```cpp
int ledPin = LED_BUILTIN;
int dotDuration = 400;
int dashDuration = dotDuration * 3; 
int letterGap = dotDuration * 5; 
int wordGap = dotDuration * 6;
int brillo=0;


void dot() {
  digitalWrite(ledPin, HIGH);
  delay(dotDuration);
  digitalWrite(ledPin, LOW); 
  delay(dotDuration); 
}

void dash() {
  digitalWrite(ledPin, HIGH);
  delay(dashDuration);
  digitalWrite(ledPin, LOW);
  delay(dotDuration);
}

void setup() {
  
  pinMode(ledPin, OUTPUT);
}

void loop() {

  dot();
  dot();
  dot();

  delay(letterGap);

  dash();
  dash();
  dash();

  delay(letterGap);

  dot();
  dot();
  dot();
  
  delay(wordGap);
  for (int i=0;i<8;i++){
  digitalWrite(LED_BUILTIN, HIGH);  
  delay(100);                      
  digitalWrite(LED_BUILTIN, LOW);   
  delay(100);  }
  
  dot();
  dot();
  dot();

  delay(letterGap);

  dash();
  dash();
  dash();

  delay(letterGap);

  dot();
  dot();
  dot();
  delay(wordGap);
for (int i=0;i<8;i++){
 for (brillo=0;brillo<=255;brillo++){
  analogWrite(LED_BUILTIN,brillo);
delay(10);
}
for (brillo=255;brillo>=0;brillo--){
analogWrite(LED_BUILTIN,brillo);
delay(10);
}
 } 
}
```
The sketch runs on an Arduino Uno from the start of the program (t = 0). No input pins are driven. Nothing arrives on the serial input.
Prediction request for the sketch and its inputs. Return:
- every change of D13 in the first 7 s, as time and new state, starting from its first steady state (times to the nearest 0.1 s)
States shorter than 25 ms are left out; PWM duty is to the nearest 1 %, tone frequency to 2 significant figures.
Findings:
0 s high; 0.4 s low; 0.8 s high; 1.2 s low; 1.6 s high; 2 s low; 4.4 s high; 5.6 s low; 6 s high
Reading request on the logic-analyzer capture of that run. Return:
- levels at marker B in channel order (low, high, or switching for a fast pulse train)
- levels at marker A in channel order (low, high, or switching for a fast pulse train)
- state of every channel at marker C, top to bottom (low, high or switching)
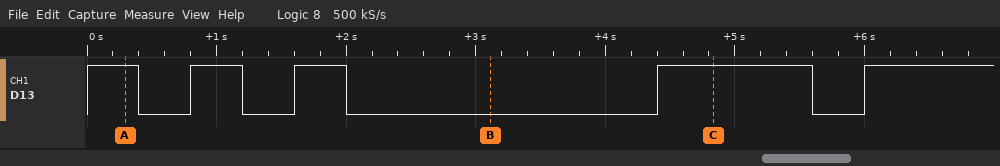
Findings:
D13 low
D13 high
D13 high
